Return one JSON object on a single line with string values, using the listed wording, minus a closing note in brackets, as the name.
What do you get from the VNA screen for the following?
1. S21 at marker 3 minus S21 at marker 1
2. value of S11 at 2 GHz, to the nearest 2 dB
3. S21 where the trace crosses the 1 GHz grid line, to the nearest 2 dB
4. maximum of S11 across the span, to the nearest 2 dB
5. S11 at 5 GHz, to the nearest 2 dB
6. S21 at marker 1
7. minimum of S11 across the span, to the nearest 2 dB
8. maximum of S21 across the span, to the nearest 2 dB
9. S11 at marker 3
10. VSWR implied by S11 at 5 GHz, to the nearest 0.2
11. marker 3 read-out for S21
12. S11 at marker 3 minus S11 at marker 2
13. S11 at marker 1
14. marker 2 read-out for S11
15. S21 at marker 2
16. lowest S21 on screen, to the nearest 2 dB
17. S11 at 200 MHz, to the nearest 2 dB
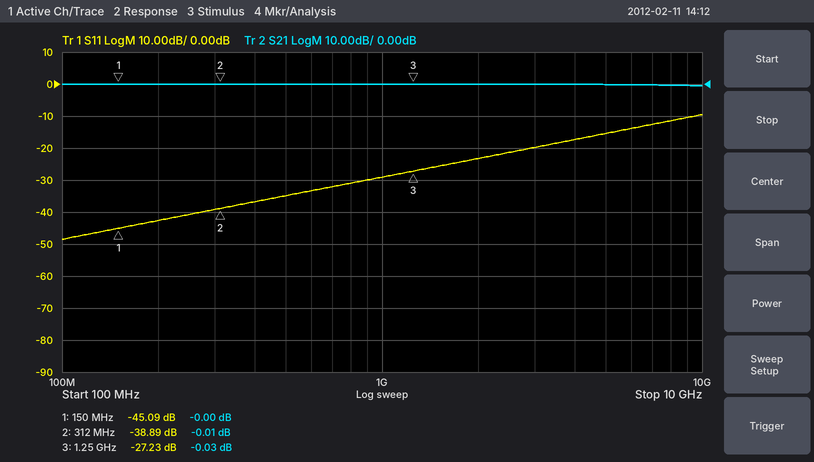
{"S21 at marker 3 minus S21 at marker 1": "-0.03 dB", "value of S11 at 2 GHz, to the nearest 2 dB": "-24 dB", "S21 where the trace crosses the 1 GHz grid line, to the nearest 2 dB": "0 dB", "maximum of S11 across the span, to the nearest 2 dB": "-10 dB", "S11 at 5 GHz, to the nearest 2 dB": "-16 dB", "S21 at marker 1": "-0.00 dB", "minimum of S11 across the span, to the nearest 2 dB": "-48 dB", "maximum of S21 across the span, to the nearest 2 dB": "0 dB", "S11 at marker 3": "-27.23 dB", "VSWR implied by S11 at 5 GHz, to the nearest 0.2": "1.4", "marker 3 read-out for S21": "-0.03 dB", "S11 at marker 3 minus S11 at marker 2": "11.66 dB", "S11 at marker 1": "-45.09 dB", "marker 2 read-out for S11": "-38.89 dB", "S21 at marker 2": "-0.01 dB", "lowest S21 on screen, to the nearest 2 dB": "0 dB", "S11 at 200 MHz, to the nearest 2 dB": "-42 dB"}
